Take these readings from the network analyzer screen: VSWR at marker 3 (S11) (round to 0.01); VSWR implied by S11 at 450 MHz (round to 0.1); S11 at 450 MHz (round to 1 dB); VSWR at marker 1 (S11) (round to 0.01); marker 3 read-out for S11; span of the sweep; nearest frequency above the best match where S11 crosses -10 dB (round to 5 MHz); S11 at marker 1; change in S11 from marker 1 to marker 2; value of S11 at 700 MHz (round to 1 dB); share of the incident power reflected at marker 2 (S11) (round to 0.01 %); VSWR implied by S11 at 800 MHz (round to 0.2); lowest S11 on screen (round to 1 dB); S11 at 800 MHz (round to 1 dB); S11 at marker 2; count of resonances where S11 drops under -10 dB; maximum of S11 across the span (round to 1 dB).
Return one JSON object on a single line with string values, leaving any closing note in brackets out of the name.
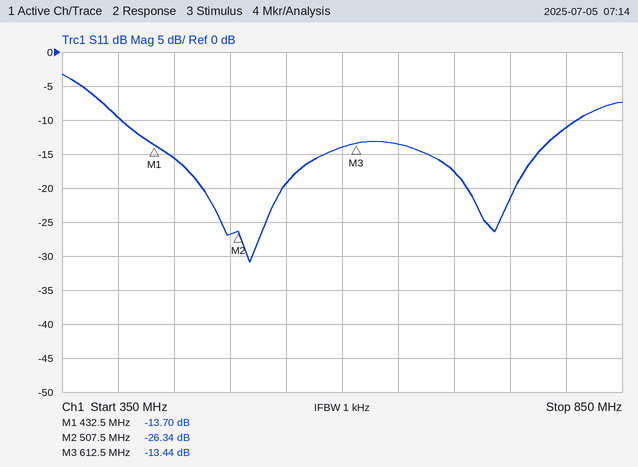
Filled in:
{"VSWR at marker 3 (S11)": "1.54", "VSWR implied by S11 at 450 MHz": "1.4", "S11 at 450 MHz": "-16 dB", "VSWR at marker 1 (S11)": "1.52", "marker 3 read-out for S11": "-13.44 dB", "span of the sweep": "500 MHz", "nearest frequency above the best match where S11 crosses -10 dB": "810 MHz", "S11 at marker 1": "-13.70 dB", "change in S11 from marker 1 to marker 2": "-12.64 dB", "value of S11 at 700 MHz": "-18 dB", "share of the incident power reflected at marker 2 (S11)": "0.23 %", "VSWR implied by S11 at 800 MHz": "1.8", "lowest S11 on screen": "-31 dB", "S11 at 800 MHz": "-11 dB", "S11 at marker 2": "-26.34 dB", "count of resonances where S11 drops under -10 dB": "2", "maximum of S11 across the span": "-3 dB"}
